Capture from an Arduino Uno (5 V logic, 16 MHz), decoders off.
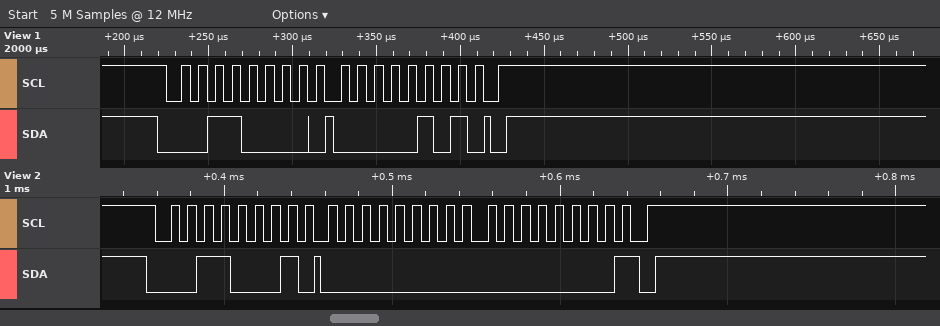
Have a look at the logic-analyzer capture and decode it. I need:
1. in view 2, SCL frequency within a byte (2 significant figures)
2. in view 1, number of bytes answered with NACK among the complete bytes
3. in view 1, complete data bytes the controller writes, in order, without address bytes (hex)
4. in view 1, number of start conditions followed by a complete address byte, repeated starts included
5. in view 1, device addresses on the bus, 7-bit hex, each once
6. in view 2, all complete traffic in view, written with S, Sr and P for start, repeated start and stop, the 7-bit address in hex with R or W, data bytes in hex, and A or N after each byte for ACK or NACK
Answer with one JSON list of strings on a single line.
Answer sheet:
["100 kHz", "0", "05", "1", "0x18", "S 18R A 00 A 00 N P"]
